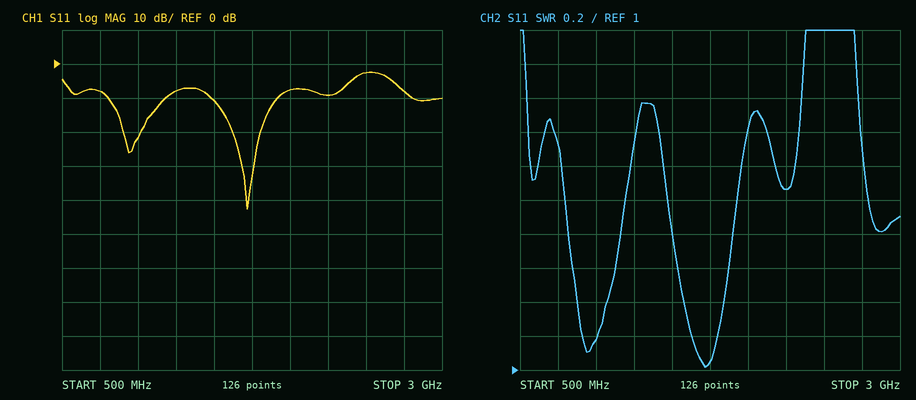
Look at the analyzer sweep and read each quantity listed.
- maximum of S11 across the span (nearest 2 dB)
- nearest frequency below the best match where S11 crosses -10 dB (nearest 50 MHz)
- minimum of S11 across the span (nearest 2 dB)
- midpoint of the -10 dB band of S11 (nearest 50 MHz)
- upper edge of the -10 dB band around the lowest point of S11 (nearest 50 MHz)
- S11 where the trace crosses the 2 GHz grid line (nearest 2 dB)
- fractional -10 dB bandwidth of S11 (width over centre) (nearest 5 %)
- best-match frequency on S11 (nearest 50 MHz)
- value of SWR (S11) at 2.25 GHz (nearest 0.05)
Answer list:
-2 dB
1.50 GHz
-42 dB
1.70 GHz
1.90 GHz
-8 dB
25 %
1.70 GHz
2.05
